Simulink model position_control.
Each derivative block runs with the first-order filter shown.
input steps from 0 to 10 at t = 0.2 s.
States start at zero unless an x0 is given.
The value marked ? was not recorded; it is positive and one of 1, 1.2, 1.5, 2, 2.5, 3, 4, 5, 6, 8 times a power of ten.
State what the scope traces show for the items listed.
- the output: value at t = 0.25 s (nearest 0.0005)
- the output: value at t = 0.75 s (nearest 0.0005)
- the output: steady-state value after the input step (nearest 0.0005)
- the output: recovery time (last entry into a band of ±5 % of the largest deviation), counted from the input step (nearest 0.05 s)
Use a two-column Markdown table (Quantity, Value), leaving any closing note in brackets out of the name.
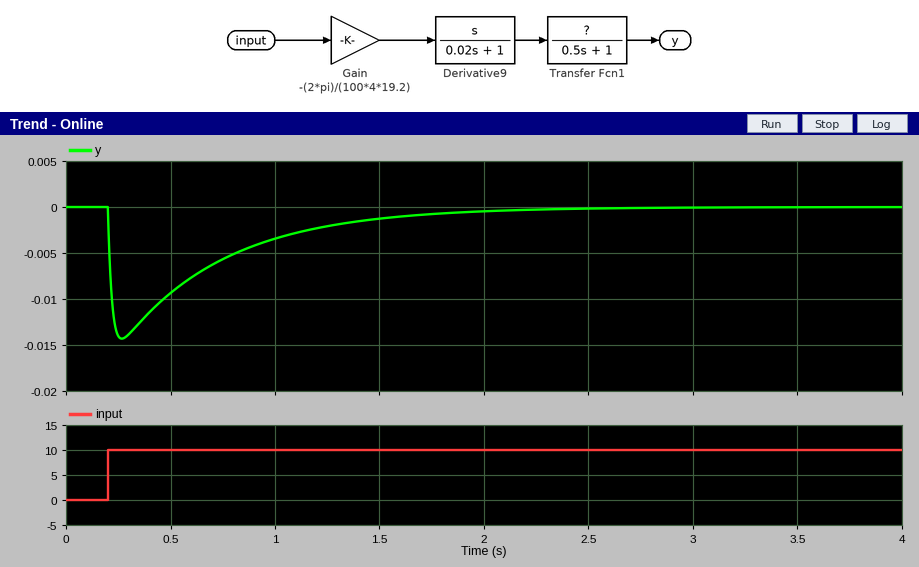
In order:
| Quantity | Value |
|---|---|
| the output: value at t = 0.25 s | -0.0140 |
| the output: value at t = 0.75 s | -0.0055 |
| the output: steady-state value after the input step | 0.0000 |
| the output: recovery time (last entry into a band of ±5 % of the largest deviation), counted from the input step | 1.60 s |
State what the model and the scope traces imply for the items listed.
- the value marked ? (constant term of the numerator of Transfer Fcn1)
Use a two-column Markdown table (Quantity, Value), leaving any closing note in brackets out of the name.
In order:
| Quantity | Value |
|---|---|
| the value marked ? | 1 |
